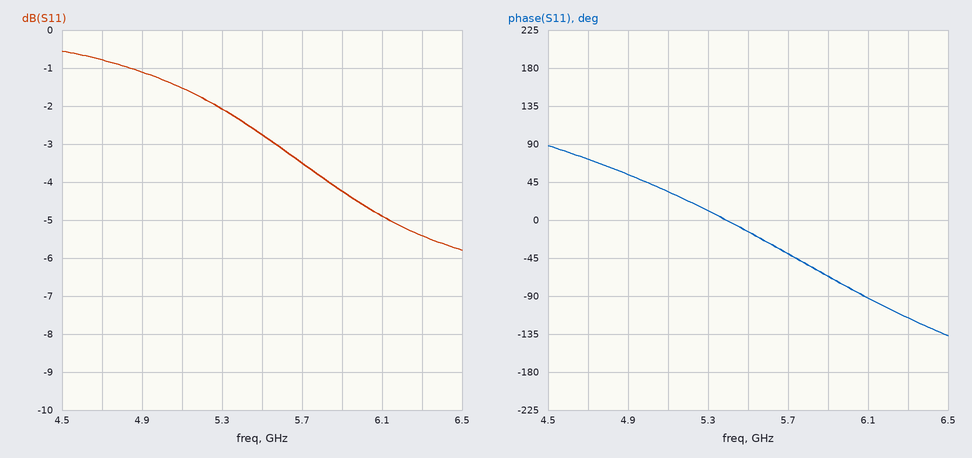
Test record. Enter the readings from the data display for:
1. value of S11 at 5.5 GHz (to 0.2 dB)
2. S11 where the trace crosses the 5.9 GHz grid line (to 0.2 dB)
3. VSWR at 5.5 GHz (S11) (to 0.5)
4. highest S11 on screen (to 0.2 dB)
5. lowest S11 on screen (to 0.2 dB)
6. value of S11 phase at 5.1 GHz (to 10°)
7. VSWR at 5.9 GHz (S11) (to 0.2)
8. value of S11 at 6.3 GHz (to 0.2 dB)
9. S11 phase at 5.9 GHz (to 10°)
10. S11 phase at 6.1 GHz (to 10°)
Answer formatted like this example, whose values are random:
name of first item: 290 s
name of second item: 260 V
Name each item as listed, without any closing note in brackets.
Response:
value of S11 at 5.5 GHz: -2.8 dB
S11 where the trace crosses the 5.9 GHz grid line: -4.2 dB
VSWR at 5.5 GHz (S11): 6.5
highest S11 on screen: -0.6 dB
lowest S11 on screen: -5.8 dB
value of S11 phase at 5.1 GHz: 30°
VSWR at 5.9 GHz (S11): 4.2
value of S11 at 6.3 GHz: -5.4 dB
S11 phase at 5.9 GHz: -70°
S11 phase at 6.1 GHz: -90°
